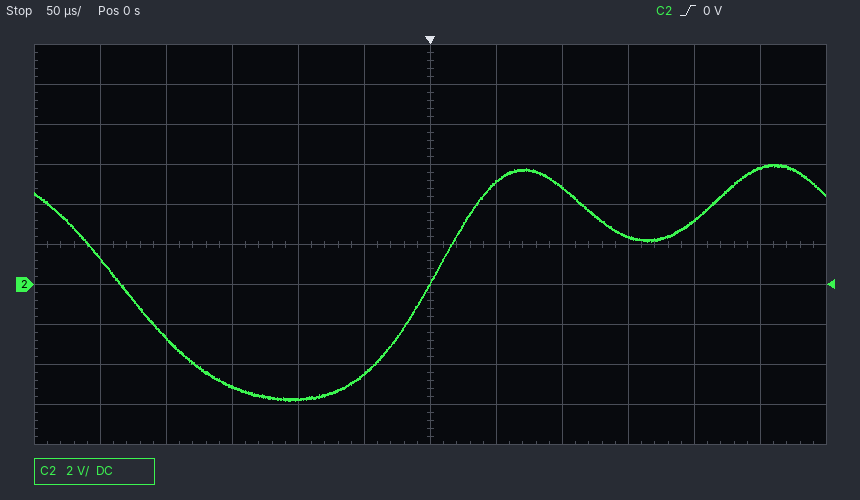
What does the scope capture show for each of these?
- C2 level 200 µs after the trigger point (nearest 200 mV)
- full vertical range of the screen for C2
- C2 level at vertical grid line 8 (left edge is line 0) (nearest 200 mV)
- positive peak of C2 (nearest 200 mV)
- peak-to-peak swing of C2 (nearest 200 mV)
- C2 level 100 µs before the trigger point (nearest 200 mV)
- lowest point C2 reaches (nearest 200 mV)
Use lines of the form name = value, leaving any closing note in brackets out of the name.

C2 level 200 µs after the trigger point = 3.2 V
full vertical range of the screen for C2 = 20 V
C2 level at vertical grid line 8 (left edge is line 0) = 4.8 V
positive peak of C2 = 6.0 V
peak-to-peak swing of C2 = 11.8 V
C2 level 100 µs before the trigger point = -5.8 V
lowest point C2 reaches = -5.8 V
